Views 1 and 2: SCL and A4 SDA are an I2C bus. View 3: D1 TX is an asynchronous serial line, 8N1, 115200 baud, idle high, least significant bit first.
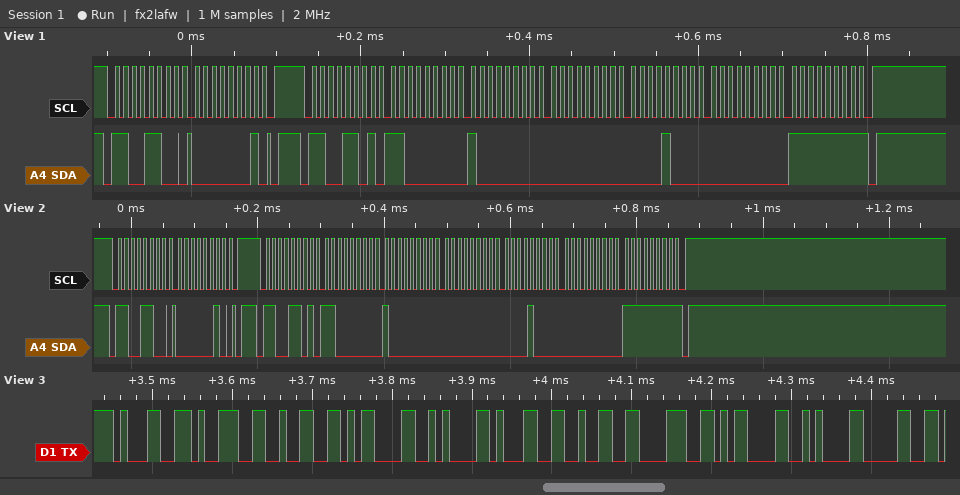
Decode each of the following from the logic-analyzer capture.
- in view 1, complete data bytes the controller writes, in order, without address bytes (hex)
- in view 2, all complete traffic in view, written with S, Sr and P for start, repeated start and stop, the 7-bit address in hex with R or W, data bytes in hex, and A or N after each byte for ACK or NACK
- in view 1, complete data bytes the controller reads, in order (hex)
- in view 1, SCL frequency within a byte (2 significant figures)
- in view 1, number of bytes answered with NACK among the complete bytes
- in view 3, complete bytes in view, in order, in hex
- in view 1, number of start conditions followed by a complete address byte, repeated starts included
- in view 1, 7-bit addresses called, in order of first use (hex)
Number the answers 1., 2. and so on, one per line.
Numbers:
1. 01
2. S 66W A 02 A P S 66R A C0 A 80 A 00 A 08 A 00 A FF N P
3. C0 80 00 08 00 FF
4. 100 kHz
5. 1
6. 31 39 32 0D 0A 31 32 38 0D 0A 30
7. 2
8. 0x66
